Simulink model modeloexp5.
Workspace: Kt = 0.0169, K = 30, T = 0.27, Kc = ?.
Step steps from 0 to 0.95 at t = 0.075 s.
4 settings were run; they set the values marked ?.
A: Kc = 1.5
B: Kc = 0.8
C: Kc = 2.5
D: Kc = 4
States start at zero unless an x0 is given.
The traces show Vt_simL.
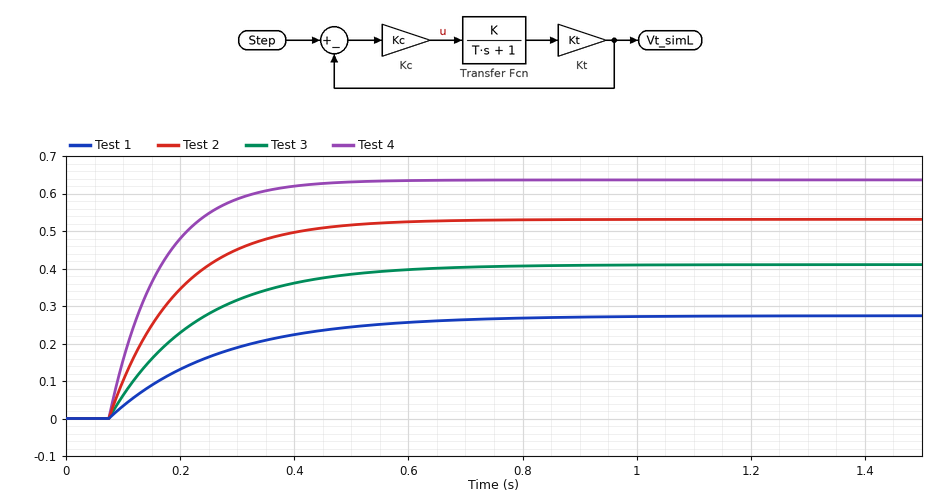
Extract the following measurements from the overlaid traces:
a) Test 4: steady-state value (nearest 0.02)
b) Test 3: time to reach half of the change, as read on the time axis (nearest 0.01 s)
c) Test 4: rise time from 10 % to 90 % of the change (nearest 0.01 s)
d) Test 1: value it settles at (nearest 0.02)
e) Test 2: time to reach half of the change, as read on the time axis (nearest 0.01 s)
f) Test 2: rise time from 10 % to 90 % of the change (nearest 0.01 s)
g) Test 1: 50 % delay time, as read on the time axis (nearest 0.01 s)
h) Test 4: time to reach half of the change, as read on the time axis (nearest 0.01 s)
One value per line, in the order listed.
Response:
0.64
0.18 s
0.20 s
0.28
0.16 s
0.26 s
0.21 s
0.14 s
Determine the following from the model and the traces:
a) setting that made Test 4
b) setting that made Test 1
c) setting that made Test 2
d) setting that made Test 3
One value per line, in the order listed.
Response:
D
B
C
A
